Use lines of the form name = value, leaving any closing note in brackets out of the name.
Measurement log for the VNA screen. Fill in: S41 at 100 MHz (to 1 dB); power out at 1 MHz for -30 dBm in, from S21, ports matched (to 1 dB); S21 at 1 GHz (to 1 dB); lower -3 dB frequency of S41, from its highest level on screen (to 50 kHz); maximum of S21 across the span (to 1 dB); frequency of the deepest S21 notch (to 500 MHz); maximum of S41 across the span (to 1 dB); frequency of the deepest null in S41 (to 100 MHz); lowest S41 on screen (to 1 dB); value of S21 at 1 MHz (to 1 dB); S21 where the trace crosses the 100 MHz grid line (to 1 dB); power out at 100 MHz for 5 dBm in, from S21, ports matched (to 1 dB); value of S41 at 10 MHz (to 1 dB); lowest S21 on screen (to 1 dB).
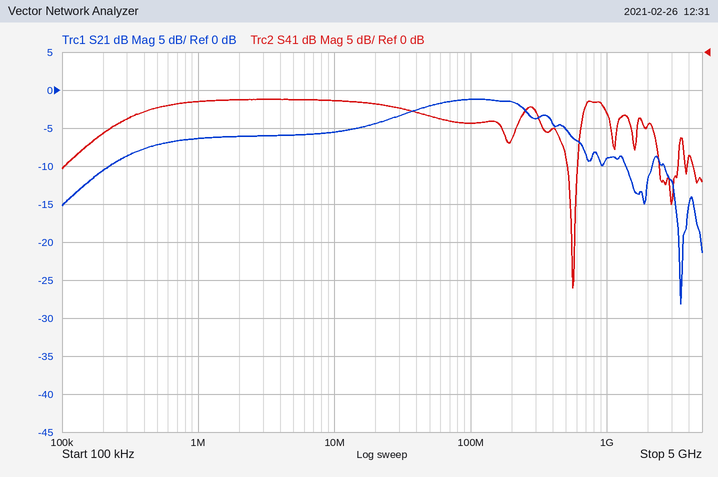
S41 at 100 MHz = -9 dB
power out at 1 MHz for -30 dBm in, from S21, ports matched = -36 dBm
S21 at 1 GHz = -9 dB
lower -3 dB frequency of S41, from its highest level on screen = 250 kHz
maximum of S21 across the span = -1 dB
frequency of the deepest S21 notch = 3.5 GHz
maximum of S41 across the span = -6 dB
frequency of the deepest null in S41 = 600 MHz
lowest S41 on screen = -31 dB
value of S21 at 1 MHz = -6 dB
S21 where the trace crosses the 100 MHz grid line = -1 dB
power out at 100 MHz for 5 dBm in, from S21, ports matched = 4 dBm
value of S41 at 10 MHz = -6 dB
lowest S21 on screen = -28 dB
